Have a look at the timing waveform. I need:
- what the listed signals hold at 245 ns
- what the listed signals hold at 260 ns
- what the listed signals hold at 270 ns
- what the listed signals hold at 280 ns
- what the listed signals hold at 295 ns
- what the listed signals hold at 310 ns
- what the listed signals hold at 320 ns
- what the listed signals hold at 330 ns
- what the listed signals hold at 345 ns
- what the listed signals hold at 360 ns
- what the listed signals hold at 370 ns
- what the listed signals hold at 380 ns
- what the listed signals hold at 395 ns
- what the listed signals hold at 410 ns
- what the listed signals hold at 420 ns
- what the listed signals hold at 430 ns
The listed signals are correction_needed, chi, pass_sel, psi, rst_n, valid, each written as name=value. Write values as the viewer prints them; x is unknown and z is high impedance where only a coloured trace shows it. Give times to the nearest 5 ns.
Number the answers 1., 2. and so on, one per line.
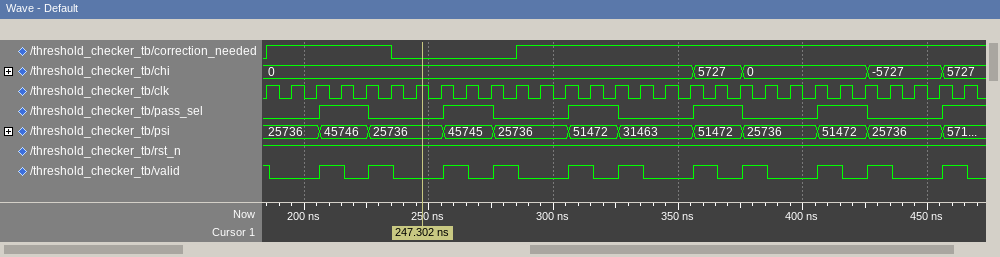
1. correction_needed=0, chi=0, pass_sel=0, psi=25736, rst_n=1, valid=0
2. correction_needed=0, chi=0, pass_sel=1, psi=45745, rst_n=1, valid=1
3. correction_needed=0, chi=0, pass_sel=1, psi=45745, rst_n=1, valid=0
4. correction_needed=0, chi=0, pass_sel=0, psi=25736, rst_n=1, valid=1
5. correction_needed=1, chi=0, pass_sel=0, psi=25736, rst_n=1, valid=0
6. correction_needed=1, chi=0, pass_sel=1, psi=51472, rst_n=1, valid=1
7. correction_needed=1, chi=0, pass_sel=1, psi=51472, rst_n=1, valid=0
8. correction_needed=1, chi=0, pass_sel=0, psi=31463, rst_n=1, valid=1
9. correction_needed=1, chi=0, pass_sel=0, psi=31463, rst_n=1, valid=0
10. correction_needed=1, chi=5727, pass_sel=1, psi=51472, rst_n=1, valid=1
11. correction_needed=1, chi=5727, pass_sel=1, psi=51472, rst_n=1, valid=0
12. correction_needed=1, chi=0, pass_sel=0, psi=25736, rst_n=1, valid=1
13. correction_needed=1, chi=0, pass_sel=0, psi=25736, rst_n=1, valid=0
14. correction_needed=1, chi=0, pass_sel=1, psi=51472, rst_n=1, valid=1
15. correction_needed=1, chi=0, pass_sel=1, psi=51472, rst_n=1, valid=0
16. correction_needed=1, chi=-5727, pass_sel=0, psi=25736, rst_n=1, valid=1
